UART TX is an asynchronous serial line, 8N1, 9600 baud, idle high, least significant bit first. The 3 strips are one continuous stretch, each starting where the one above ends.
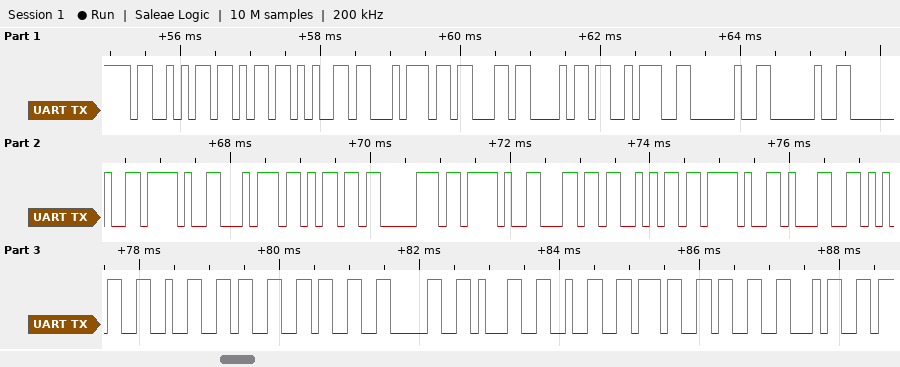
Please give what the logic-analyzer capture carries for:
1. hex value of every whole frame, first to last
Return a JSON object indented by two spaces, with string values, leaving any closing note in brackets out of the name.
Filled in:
{
  "hex value of every whole frame, first to last": "53 6B 65 74 63 68 3A 20 20 20 2F 74 6D 70 2F 6C 6A 2F 31 35 32 33 33 30 31 32 37 33 34"
}
